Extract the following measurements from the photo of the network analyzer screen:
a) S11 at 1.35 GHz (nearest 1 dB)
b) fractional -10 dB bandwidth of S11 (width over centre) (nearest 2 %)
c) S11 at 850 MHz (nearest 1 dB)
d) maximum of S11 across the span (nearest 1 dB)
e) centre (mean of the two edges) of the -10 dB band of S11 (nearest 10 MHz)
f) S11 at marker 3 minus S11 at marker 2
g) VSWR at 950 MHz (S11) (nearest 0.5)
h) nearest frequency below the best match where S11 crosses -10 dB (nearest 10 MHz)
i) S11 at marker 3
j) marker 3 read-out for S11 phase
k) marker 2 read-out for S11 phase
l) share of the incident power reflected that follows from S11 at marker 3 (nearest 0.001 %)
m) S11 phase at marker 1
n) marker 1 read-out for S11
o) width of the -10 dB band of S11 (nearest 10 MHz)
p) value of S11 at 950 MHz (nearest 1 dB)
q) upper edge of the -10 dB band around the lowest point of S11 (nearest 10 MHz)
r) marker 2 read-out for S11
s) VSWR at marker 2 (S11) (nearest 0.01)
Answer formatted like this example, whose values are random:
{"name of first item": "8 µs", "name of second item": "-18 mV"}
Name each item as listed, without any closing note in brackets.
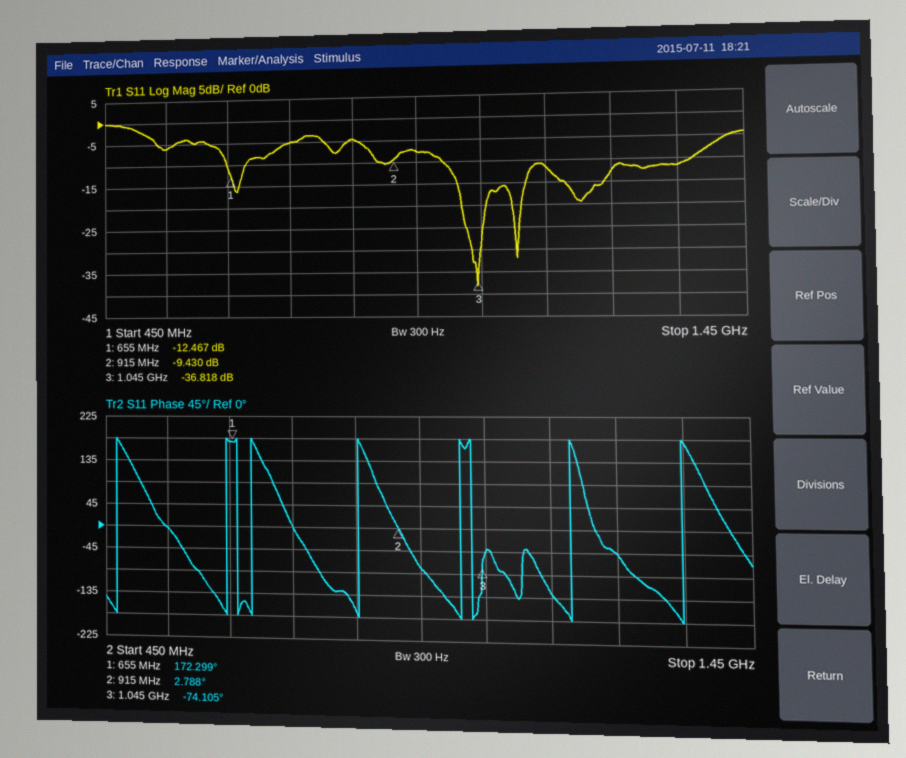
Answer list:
{"S11 at 1.35 GHz": "-12 dB", "fractional -10 dB bandwidth of S11 (width over centre)": "32 %", "S11 at 850 MHz": "-5 dB", "maximum of S11 across the span": "0 dB", "centre (mean of the two edges) of the -10 dB band of S11": "1.18 GHz", "S11 at marker 3 minus S11 at marker 2": "-27.388 dB", "VSWR at 950 MHz (S11)": "2.5", "nearest frequency below the best match where S11 crosses -10 dB": "990 MHz", "S11 at marker 3": "-36.818 dB", "marker 3 read-out for S11 phase": "-74.105°", "marker 2 read-out for S11 phase": "2.788°", "share of the incident power reflected that follows from S11 at marker 3": "0.021 %", "S11 phase at marker 1": "172.299°", "marker 1 read-out for S11": "-12.467 dB", "width of the -10 dB band of S11": "380 MHz", "value of S11 at 950 MHz": "-8 dB", "upper edge of the -10 dB band around the lowest point of S11": "1.37 GHz", "marker 2 read-out for S11": "-9.430 dB", "VSWR at marker 2 (S11)": "2.02"}
